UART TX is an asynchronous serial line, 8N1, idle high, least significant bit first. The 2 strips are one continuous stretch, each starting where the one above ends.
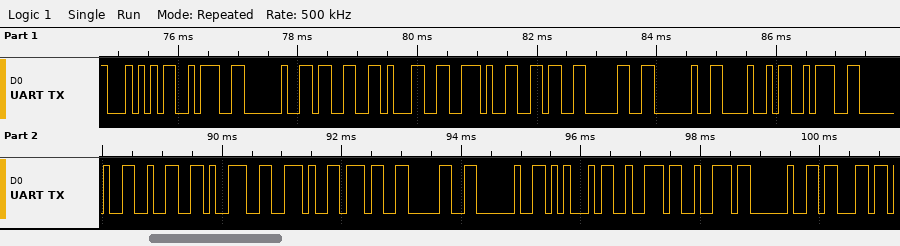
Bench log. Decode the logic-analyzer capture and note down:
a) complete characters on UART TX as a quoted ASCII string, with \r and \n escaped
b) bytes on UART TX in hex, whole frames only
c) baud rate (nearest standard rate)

"T: 31.60 H: 29.70 Err c"
54 3A 20 33 31 2E 36 30 20 48 3A 20 32 39 2E 37 30 20 45 72 72 20 63
9600 baud
